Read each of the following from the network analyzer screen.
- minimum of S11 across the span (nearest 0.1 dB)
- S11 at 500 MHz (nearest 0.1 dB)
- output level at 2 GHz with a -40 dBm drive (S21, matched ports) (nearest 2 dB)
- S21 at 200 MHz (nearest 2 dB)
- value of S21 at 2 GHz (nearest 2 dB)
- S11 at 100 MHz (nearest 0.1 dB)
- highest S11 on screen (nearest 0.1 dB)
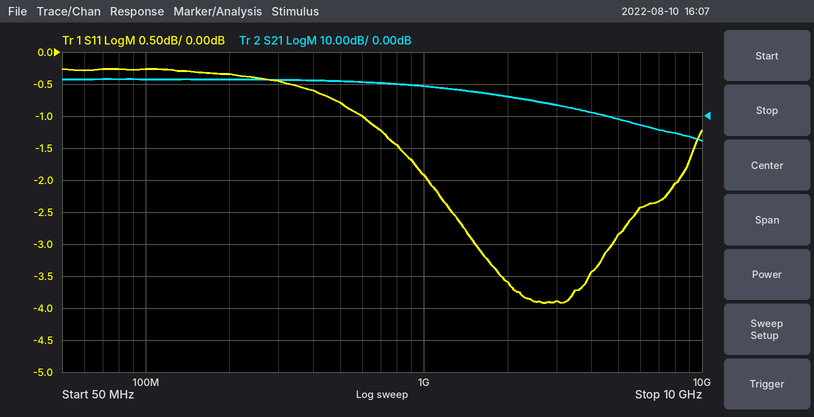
-3.9 dB
-0.8 dB
-34 dBm
12 dB
6 dB
-0.3 dB
-0.3 dB
